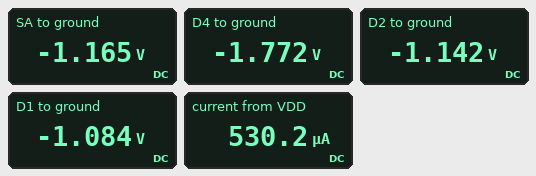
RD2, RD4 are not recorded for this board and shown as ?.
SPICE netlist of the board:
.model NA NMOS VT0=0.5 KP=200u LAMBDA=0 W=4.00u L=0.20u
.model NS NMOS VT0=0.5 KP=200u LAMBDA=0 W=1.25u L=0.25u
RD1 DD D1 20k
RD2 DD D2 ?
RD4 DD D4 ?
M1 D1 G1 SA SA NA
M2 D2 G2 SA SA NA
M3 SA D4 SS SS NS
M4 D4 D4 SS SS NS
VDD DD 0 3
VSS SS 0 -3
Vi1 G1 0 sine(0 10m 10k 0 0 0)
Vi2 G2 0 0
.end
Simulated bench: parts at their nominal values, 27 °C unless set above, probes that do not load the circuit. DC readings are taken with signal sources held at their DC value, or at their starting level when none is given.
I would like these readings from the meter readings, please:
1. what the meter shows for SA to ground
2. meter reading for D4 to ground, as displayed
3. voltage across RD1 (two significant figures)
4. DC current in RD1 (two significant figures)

-1.165 V
-1.772 V
4.1 V
200 µA
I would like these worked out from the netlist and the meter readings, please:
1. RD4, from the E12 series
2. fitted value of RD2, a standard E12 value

18 kΩ
68 kΩ
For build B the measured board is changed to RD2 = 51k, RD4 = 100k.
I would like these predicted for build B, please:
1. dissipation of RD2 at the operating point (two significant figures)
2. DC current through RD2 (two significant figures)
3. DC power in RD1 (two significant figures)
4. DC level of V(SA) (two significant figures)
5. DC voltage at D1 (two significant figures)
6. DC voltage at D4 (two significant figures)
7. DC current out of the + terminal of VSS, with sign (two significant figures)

34 µW
26 µA
13 µW
-610 mV
2.5 V
-2.2 V
-100 µA
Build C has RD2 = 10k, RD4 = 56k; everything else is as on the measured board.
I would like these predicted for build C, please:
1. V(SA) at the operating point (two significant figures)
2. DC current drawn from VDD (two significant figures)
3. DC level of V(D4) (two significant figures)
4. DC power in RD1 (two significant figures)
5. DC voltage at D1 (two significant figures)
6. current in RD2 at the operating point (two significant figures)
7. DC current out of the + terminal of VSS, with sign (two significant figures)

-650 mV
180 µA
-2.1 V
41 µW
2.1 V
45 µA
-180 µA
